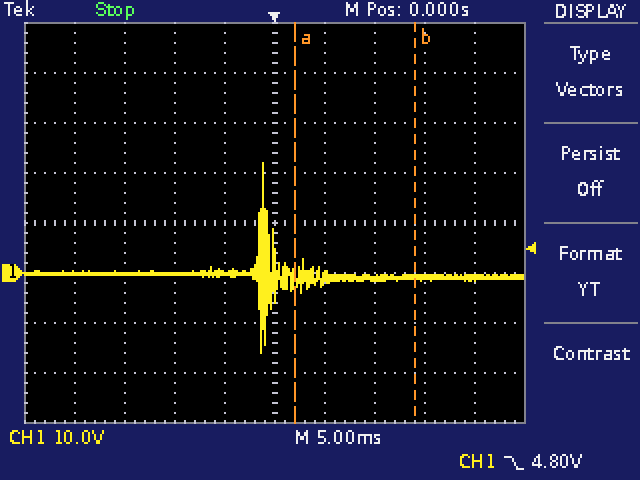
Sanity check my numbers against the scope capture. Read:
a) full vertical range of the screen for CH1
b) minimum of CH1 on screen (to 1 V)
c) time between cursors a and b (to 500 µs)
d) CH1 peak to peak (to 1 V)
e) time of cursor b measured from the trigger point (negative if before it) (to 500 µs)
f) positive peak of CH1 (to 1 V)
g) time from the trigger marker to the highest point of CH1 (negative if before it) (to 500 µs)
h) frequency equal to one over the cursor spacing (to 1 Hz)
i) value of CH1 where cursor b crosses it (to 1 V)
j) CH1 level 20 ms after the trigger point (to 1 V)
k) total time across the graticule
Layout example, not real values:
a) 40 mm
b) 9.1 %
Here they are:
a) 80 V
b) -16 V
c) 12.0 ms
d) 38 V
e) +14.0 ms
f) 22 V
g) -1.0 ms
h) 83 Hz
i) -1 V
j) -1 V
k) 50 ms
